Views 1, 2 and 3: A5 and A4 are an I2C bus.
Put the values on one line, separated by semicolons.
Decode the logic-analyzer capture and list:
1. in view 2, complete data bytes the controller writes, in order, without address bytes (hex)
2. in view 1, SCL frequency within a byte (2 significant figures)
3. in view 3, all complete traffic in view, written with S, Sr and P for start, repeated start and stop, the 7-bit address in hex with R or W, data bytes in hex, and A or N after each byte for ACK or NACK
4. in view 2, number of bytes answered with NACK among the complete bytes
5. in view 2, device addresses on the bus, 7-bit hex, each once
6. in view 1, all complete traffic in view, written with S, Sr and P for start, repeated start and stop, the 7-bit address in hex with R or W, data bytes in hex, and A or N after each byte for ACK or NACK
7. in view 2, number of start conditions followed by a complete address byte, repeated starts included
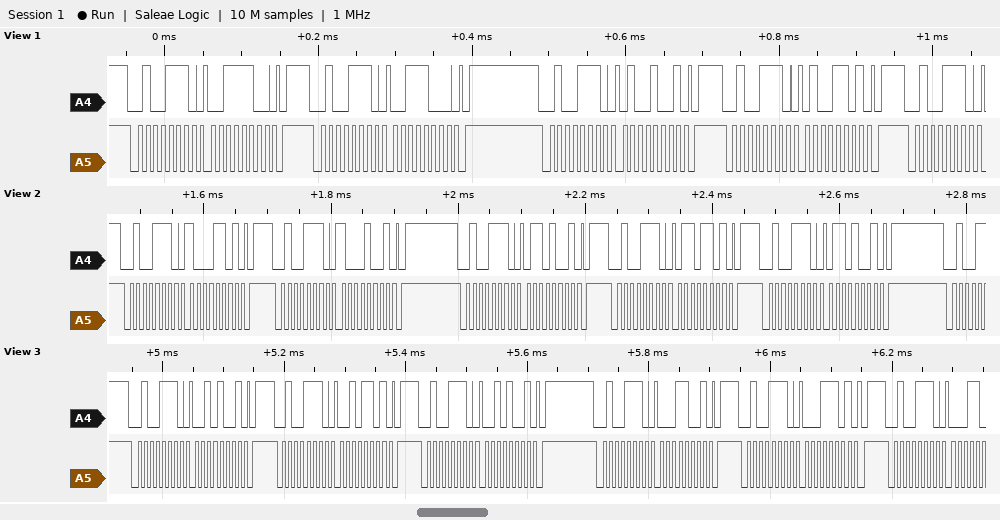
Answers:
8D 89 69 6D 69; 100 kHz; S 27W A 29 A P S 27W A 2D A P S 27W A 29 A P S 27W A 19 A P S 27W A 1D A P S 27W A; 0; 0x27; S 27W A 3C A P S 27W A 38 A P S 27W A 49 A P S 27W A 4D A P S 27W A; 5
